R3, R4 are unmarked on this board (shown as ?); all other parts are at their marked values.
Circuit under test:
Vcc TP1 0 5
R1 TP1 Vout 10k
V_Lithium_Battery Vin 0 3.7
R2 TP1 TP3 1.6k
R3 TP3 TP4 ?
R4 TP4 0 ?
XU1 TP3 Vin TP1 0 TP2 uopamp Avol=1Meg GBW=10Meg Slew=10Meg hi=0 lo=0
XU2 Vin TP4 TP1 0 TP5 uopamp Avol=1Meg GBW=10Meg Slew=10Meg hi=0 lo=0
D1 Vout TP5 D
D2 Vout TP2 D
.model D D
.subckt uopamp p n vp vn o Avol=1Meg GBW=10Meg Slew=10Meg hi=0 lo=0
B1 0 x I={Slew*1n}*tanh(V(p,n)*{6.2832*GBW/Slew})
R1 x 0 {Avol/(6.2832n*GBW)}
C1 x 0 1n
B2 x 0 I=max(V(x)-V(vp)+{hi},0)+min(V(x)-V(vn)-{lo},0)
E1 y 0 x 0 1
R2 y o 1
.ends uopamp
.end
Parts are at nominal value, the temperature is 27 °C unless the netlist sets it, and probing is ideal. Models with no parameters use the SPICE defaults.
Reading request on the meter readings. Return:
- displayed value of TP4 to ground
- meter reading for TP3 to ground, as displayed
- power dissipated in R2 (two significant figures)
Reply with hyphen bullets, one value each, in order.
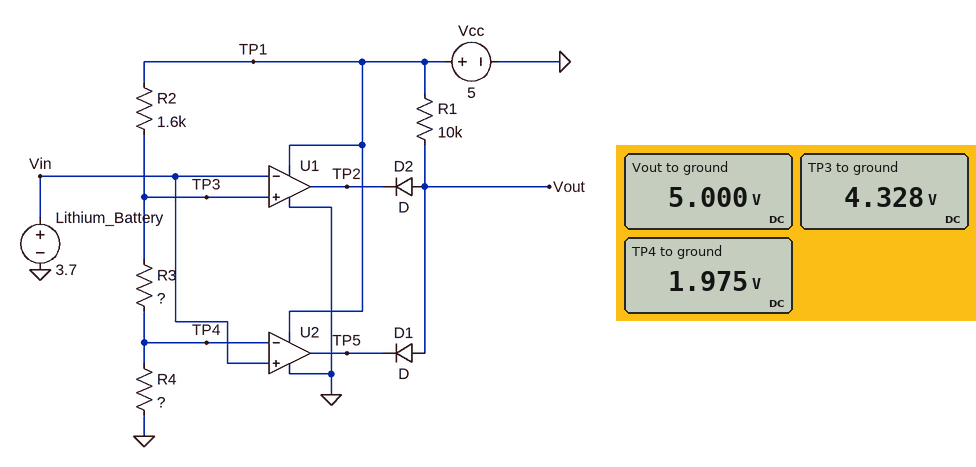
- 1.975 V
- 4.328 V
- 280 µW
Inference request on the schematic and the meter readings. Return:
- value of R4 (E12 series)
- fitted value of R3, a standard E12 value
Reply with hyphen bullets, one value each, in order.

- 4.7 kΩ
- 5.6 kΩ
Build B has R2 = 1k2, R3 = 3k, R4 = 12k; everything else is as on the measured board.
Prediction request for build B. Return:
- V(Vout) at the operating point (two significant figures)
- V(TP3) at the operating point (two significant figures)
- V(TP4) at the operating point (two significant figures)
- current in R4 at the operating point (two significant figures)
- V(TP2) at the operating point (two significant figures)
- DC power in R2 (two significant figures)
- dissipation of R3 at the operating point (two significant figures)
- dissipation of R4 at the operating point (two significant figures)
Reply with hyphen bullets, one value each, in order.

- 630 mV
- 4.6 V
- 3.7 V
- 310 µA
- 5.0 V
- 110 µW
- 290 µW
- 1.1 mW
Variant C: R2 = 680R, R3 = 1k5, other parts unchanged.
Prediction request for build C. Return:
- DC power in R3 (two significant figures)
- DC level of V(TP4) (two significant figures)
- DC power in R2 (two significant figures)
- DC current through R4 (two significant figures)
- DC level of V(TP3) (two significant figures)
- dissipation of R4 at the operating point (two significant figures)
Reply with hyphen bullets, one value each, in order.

- 790 µW
- 3.4 V
- 360 µW
- 730 µA
- 4.5 V
- 2.5 mW
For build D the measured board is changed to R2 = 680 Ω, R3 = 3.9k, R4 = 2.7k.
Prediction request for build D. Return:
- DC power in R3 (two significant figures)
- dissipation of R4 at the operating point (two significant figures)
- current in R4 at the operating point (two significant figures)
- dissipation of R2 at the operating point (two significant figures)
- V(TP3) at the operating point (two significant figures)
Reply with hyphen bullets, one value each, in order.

- 1.8 mW
- 1.3 mW
- 690 µA
- 320 µW
- 4.5 V
